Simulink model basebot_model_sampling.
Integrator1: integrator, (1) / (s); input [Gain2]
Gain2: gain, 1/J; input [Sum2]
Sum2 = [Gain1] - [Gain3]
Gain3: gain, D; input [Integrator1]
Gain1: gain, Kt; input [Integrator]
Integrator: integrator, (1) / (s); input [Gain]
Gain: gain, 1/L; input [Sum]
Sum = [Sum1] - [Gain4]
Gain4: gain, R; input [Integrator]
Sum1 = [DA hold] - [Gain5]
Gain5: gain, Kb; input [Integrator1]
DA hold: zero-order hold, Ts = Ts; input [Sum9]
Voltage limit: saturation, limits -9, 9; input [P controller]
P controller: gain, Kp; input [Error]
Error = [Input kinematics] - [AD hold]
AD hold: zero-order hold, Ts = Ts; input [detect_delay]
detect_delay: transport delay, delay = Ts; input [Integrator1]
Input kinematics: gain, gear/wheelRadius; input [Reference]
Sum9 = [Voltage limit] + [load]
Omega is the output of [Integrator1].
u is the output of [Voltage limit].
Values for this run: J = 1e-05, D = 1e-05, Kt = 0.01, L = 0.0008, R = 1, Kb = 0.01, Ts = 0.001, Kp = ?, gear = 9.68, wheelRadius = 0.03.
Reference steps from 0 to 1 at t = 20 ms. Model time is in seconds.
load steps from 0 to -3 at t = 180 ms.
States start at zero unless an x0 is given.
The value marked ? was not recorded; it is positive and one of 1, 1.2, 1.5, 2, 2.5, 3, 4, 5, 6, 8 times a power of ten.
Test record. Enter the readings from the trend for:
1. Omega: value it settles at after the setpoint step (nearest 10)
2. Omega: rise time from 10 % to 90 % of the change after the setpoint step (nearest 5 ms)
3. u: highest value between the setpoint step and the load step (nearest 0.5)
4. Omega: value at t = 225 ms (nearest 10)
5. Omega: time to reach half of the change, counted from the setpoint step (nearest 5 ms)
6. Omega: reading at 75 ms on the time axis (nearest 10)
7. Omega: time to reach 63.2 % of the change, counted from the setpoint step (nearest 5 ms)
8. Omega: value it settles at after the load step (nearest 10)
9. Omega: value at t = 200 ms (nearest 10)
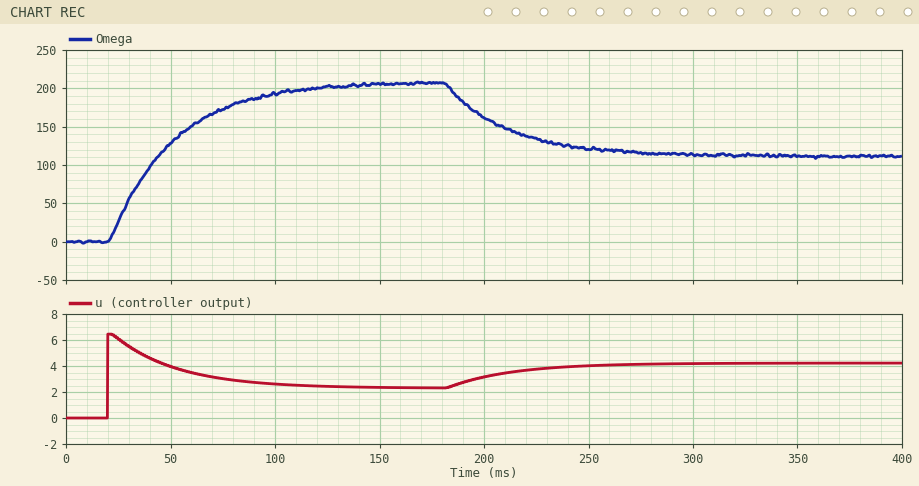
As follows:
210
65 ms
6.5
130
20 ms
170
30 ms
110
160
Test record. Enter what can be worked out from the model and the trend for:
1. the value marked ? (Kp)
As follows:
0.02
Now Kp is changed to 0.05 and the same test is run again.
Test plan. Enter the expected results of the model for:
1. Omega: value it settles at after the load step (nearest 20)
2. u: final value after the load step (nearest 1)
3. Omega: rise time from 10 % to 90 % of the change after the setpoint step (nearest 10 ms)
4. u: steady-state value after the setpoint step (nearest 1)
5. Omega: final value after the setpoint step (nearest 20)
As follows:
220
5
40 ms
3
260
